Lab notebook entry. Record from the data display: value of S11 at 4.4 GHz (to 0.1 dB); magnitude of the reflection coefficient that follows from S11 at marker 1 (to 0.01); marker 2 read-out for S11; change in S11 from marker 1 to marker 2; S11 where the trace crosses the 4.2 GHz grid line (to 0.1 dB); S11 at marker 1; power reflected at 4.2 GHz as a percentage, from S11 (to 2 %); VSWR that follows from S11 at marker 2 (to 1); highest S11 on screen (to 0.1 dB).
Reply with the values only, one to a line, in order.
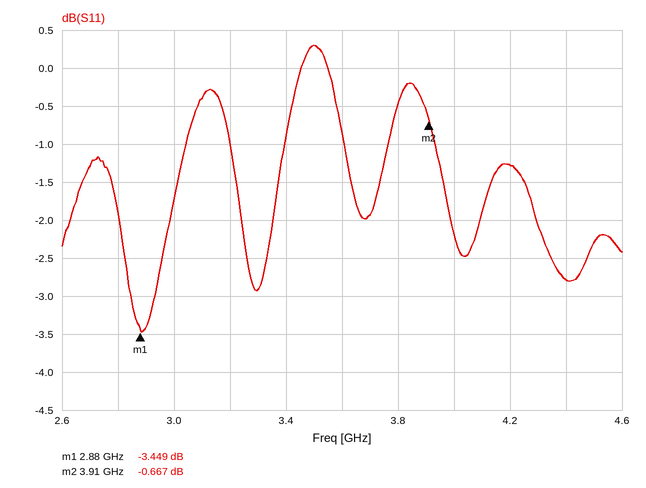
-2.8 dB
0.67
-0.667 dB
2.782 dB
-1.3 dB
-3.449 dB
74 %
26
0.3 dB
